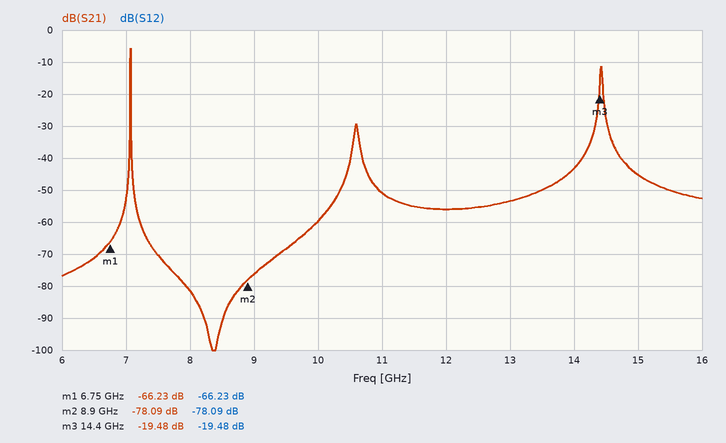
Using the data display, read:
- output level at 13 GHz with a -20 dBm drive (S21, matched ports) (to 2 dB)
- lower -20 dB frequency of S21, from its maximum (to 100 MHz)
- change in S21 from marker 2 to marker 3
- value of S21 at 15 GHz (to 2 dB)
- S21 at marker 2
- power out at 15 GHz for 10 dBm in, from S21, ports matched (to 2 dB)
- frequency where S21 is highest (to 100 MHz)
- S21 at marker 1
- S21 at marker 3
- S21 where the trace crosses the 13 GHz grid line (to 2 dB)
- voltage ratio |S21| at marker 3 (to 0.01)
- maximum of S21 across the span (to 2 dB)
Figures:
-74 dBm
7.1 GHz
58.61 dB
-46 dB
-78.09 dB
-36 dBm
7.1 GHz
-66.23 dB
-19.48 dB
-54 dB
0.11
-6 dB
